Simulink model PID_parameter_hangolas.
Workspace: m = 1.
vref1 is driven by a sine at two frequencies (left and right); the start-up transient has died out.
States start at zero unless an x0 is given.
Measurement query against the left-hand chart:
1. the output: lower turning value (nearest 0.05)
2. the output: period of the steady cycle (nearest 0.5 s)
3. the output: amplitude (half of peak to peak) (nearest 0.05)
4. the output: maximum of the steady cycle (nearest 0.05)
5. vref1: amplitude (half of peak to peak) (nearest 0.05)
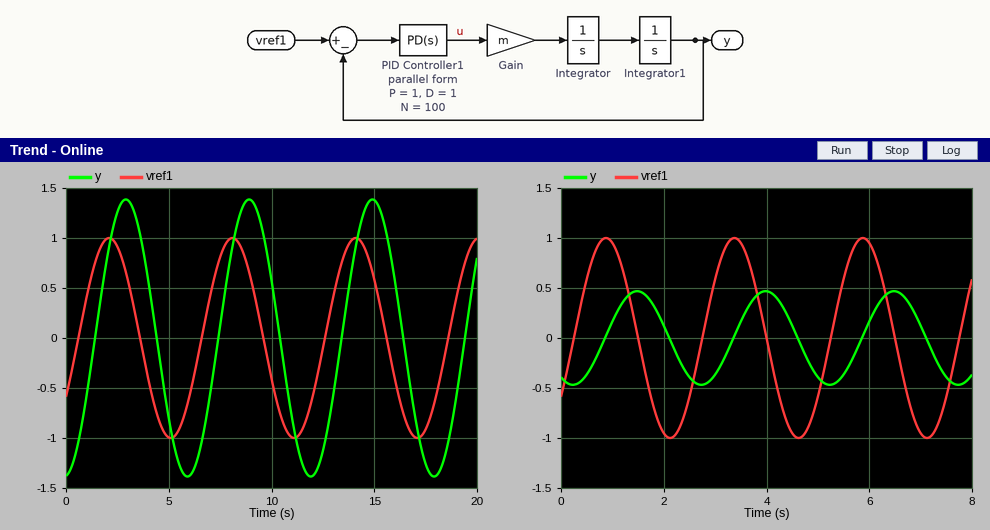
-1.40
6.0 s
1.40
1.40
1.00
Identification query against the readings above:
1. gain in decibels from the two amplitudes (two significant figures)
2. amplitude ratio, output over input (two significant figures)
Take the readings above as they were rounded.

2.9 dB
1.4
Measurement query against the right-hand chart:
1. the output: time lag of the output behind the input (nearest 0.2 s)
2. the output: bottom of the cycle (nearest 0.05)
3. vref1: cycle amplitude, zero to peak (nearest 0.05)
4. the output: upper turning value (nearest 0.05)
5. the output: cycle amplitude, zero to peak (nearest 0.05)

0.6 s
-0.45
1.00
0.45
0.45
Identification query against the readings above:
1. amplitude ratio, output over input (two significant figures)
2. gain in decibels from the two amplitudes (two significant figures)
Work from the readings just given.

0.45
-6.9 dB
